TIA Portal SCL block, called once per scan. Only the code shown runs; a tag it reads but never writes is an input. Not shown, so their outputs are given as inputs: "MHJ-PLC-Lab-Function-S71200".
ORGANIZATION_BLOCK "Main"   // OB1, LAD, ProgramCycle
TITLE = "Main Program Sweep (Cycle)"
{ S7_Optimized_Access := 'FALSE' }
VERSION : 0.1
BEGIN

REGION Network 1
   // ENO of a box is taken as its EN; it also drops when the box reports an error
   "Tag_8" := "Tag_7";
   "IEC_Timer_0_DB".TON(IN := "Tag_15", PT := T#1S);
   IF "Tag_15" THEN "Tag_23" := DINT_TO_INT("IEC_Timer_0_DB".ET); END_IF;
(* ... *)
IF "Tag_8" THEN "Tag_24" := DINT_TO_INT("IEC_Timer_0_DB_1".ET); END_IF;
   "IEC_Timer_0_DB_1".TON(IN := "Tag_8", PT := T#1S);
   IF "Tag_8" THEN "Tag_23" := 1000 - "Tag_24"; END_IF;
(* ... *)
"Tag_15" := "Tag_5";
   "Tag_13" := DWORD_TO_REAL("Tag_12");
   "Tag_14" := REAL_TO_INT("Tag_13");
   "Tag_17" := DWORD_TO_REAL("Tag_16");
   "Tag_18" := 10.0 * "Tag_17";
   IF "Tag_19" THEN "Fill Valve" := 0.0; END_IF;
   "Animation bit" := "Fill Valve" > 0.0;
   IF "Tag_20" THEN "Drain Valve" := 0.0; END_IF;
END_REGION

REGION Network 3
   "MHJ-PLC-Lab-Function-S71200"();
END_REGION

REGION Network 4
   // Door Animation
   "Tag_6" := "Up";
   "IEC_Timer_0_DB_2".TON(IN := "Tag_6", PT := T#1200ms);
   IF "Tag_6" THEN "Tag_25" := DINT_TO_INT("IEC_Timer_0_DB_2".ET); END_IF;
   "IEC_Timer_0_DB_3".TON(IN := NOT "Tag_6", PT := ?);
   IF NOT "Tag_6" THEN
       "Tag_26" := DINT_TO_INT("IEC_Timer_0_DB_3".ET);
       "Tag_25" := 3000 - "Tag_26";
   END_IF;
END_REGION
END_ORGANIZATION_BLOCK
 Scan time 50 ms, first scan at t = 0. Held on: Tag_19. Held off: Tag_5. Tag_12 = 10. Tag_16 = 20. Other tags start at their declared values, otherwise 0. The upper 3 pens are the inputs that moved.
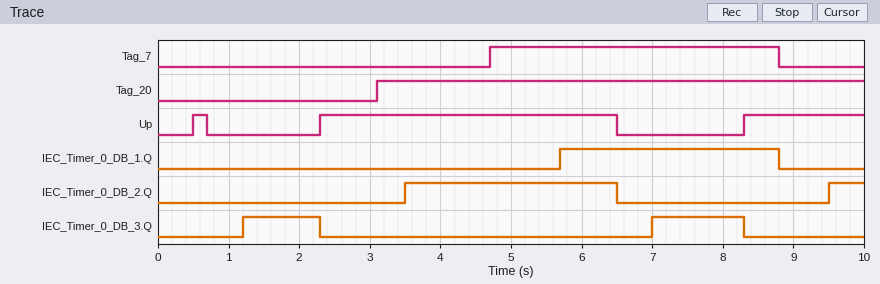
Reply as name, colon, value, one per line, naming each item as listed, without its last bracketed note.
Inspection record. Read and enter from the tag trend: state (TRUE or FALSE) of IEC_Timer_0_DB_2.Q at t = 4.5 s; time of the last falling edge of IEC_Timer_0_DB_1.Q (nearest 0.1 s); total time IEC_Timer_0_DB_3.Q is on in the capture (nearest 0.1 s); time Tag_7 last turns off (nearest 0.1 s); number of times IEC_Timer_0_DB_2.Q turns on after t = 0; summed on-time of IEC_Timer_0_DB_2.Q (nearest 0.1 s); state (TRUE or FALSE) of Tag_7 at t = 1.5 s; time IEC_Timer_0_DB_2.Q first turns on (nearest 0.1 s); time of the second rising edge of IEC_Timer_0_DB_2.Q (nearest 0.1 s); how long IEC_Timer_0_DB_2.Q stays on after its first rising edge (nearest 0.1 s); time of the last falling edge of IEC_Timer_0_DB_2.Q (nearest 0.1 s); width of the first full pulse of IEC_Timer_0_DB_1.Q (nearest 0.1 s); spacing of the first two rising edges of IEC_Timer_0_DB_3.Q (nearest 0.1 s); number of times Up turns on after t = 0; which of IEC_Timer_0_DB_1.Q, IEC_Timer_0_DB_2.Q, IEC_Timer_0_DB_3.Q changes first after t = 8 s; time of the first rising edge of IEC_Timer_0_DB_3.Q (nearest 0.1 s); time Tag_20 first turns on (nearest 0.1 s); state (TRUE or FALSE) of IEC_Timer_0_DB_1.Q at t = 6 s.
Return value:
state (TRUE or FALSE) of IEC_Timer_0_DB_2.Q at t = 4.5 s: TRUE
time of the last falling edge of IEC_Timer_0_DB_1.Q: 8.8 s
total time IEC_Timer_0_DB_3.Q is on in the capture: 2.4 s
time Tag_7 last turns off: 8.8 s
number of times IEC_Timer_0_DB_2.Q turns on after t = 0: 2
summed on-time of IEC_Timer_0_DB_2.Q: 3.5 s
state (TRUE or FALSE) of Tag_7 at t = 1.5 s: FALSE
time IEC_Timer_0_DB_2.Q first turns on: 3.5 s
time of the second rising edge of IEC_Timer_0_DB_2.Q: 9.5 s
how long IEC_Timer_0_DB_2.Q stays on after its first rising edge: 3.0 s
time of the last falling edge of IEC_Timer_0_DB_2.Q: 6.5 s
width of the first full pulse of IEC_Timer_0_DB_1.Q: 3.1 s
spacing of the first two rising edges of IEC_Timer_0_DB_3.Q: 5.8 s
number of times Up turns on after t = 0: 3
which of IEC_Timer_0_DB_1.Q, IEC_Timer_0_DB_2.Q, IEC_Timer_0_DB_3.Q changes first after t = 8 s: IEC_Timer_0_DB_3.Q
time of the first rising edge of IEC_Timer_0_DB_3.Q: 1.2 s
time Tag_20 first turns on: 3.1 s
state (TRUE or FALSE) of IEC_Timer_0_DB_1.Q at t = 6 s: TRUE
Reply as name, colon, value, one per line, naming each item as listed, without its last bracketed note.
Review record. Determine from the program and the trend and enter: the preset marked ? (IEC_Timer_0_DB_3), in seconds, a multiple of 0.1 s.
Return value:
the preset marked ? (IEC_Timer_0_DB_3), in seconds, a multiple of 0.1 s: 0.5 s
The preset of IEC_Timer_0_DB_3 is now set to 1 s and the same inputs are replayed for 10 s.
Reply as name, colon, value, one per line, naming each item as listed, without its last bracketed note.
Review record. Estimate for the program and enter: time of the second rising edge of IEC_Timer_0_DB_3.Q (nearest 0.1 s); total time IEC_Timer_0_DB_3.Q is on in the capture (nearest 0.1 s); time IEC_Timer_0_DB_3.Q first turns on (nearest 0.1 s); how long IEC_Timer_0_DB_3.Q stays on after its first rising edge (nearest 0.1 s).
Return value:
time of the second rising edge of IEC_Timer_0_DB_3.Q: 7.5 s
total time IEC_Timer_0_DB_3.Q is on in the capture: 1.4 s
time IEC_Timer_0_DB_3.Q first turns on: 1.7 s
how long IEC_Timer_0_DB_3.Q stays on after its first rising edge: 0.6 s
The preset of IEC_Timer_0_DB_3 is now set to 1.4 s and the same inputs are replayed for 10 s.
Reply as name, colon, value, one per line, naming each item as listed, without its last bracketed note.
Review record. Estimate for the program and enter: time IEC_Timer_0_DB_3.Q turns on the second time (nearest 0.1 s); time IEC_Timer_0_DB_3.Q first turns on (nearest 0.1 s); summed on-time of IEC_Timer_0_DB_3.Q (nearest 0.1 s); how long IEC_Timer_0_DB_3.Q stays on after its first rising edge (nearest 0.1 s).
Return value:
time IEC_Timer_0_DB_3.Q turns on the second time: 7.9 s
time IEC_Timer_0_DB_3.Q first turns on: 2.1 s
summed on-time of IEC_Timer_0_DB_3.Q: 0.6 s
how long IEC_Timer_0_DB_3.Q stays on after its first rising edge: 0.2 s
